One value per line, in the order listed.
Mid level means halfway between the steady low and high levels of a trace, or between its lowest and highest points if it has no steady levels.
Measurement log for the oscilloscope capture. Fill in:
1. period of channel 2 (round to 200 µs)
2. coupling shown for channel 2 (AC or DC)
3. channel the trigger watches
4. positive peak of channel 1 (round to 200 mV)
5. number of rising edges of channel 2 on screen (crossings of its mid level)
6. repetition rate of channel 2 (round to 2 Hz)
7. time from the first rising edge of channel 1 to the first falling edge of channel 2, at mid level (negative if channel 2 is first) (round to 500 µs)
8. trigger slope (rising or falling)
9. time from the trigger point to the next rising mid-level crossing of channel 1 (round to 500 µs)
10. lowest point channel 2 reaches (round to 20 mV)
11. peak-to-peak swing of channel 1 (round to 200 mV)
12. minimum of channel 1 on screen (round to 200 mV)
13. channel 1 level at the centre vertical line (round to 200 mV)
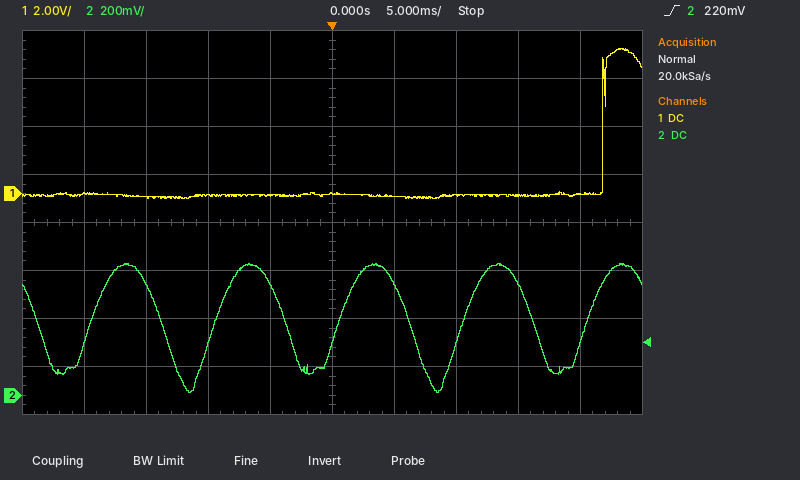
10.0 ms
DC
channel 2
6.0 V
5
100 Hz
-45.5 ms
rising
22.0 ms
20 mV
6.2 V
-200 mV
0.0 V
